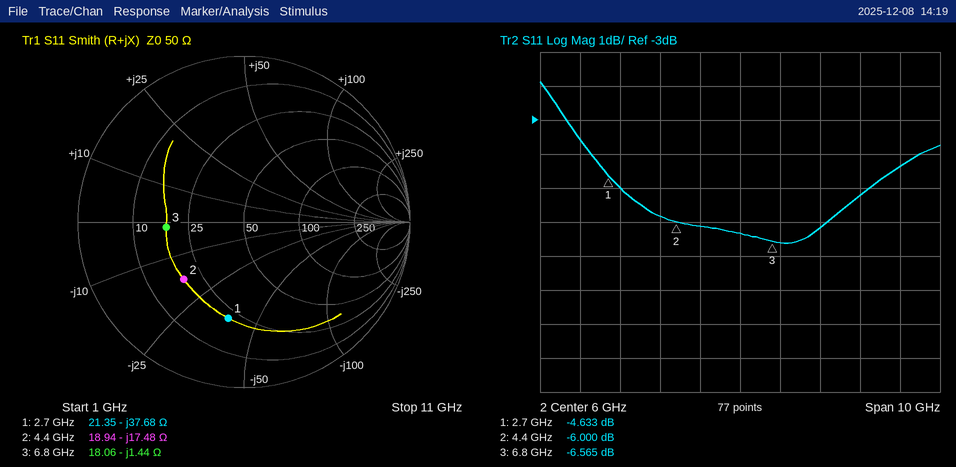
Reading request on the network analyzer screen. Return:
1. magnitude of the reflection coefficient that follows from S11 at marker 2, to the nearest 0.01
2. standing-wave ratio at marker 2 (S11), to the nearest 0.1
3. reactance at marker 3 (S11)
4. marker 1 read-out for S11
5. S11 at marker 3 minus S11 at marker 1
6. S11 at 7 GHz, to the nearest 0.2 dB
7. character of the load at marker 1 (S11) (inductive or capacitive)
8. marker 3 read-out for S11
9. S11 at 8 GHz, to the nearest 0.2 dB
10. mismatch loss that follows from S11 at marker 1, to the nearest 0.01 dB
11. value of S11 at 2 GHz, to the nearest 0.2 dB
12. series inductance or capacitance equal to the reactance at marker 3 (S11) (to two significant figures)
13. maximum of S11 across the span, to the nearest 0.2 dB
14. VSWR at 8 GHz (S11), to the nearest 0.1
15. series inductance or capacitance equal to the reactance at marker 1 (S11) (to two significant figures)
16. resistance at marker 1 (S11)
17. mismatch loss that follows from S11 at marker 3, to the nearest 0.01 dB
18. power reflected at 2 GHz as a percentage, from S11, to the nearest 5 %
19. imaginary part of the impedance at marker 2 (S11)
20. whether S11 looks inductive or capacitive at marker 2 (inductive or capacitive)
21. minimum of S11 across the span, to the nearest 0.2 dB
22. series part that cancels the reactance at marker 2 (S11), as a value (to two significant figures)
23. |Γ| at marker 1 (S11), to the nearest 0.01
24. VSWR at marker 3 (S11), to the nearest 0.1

0.50
3.0
-1.44 Ω
-4.633 dB
-1.932 dB
-6.6 dB
capacitive
-6.565 dB
-6.2 dB
1.83 dB
-3.6 dB
16 pF
-1.8 dB
2.9
1.6 pF
21.35 Ω
1.08 dB
45 %
-17.48 Ω
capacitive
-6.6 dB
630 pH
0.59
2.8
